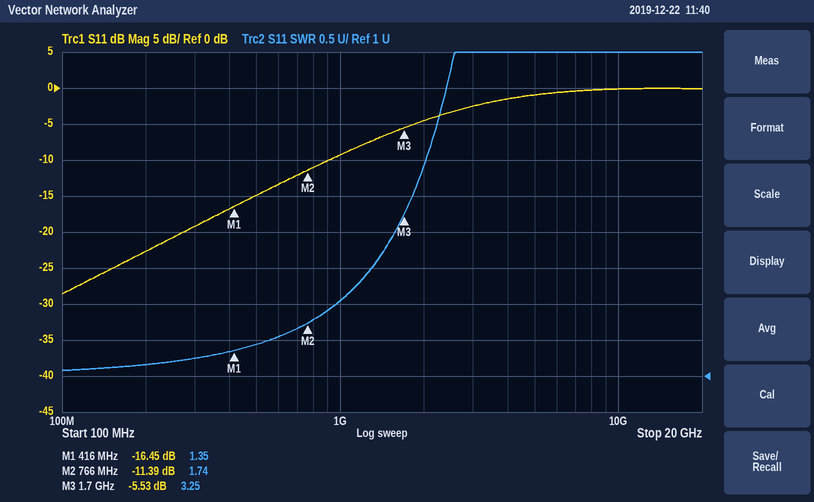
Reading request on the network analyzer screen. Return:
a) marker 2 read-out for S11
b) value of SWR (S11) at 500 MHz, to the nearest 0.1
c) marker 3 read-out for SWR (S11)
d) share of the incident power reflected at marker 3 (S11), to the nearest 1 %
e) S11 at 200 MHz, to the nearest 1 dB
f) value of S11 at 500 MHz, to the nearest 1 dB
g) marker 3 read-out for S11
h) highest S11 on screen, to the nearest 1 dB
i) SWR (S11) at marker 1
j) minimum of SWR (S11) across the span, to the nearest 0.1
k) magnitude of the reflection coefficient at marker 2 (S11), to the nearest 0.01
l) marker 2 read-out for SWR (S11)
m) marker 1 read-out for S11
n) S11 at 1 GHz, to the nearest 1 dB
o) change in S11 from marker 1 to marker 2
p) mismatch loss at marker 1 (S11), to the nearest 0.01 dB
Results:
-11.39 dB
1.4
3.25
28 %
-23 dB
-15 dB
-5.53 dB
0 dB
1.35
1.1
0.27
1.74
-16.45 dB
-9 dB
5.06 dB
0.10 dB
